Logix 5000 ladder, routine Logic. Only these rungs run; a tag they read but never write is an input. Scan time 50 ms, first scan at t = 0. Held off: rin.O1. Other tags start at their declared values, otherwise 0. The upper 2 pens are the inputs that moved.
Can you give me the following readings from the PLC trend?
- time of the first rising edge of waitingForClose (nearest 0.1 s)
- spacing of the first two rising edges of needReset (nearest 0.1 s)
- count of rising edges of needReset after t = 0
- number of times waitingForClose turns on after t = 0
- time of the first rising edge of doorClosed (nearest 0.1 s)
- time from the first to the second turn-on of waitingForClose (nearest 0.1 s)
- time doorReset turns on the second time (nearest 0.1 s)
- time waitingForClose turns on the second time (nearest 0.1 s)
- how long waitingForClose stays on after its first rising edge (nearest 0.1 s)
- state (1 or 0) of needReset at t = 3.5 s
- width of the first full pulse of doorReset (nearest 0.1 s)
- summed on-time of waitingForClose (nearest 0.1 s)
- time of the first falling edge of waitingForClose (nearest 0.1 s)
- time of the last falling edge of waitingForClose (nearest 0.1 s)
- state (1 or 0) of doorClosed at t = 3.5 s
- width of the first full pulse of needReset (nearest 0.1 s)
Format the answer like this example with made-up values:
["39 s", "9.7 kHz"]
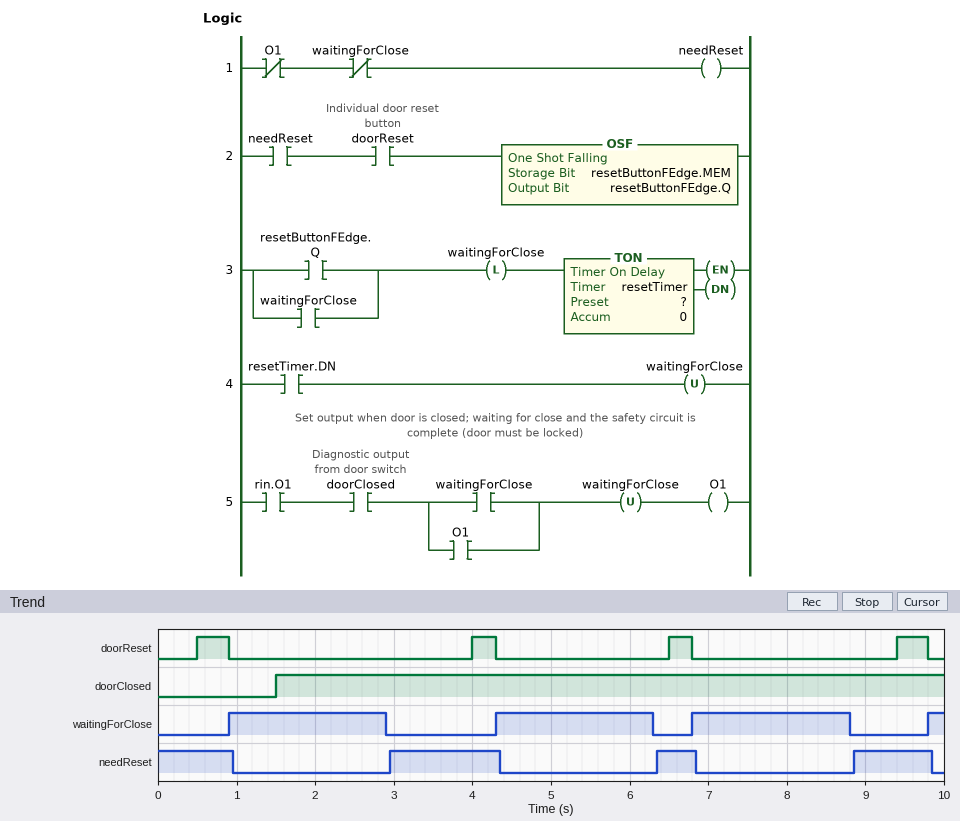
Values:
["0.9 s", "3.4 s", "3", "4", "1.5 s", "3.4 s", "4.0 s", "4.3 s", "2.0 s", "1", "0.4 s", "6.2 s", "2.9 s", "8.8 s", "1", "1.4 s"]
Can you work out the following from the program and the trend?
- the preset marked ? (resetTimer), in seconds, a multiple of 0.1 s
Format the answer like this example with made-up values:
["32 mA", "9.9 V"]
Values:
["2.0 s"]
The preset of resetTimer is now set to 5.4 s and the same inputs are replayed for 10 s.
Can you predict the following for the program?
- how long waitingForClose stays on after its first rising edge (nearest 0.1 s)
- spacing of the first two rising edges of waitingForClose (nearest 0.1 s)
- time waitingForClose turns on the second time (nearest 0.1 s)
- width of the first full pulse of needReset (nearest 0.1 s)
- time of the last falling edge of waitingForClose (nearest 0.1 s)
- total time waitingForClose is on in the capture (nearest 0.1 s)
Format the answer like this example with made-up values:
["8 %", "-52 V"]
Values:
["5.4 s", "5.9 s", "6.8 s", "0.5 s", "6.3 s", "8.6 s"]
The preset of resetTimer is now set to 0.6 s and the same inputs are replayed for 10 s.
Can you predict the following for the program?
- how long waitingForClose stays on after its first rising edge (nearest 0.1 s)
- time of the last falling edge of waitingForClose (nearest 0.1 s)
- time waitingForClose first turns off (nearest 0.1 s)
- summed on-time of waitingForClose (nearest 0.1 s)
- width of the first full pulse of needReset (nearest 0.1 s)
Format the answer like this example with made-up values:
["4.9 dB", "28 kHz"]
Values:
["0.6 s", "7.4 s", "1.5 s", "2.0 s", "2.8 s"]
